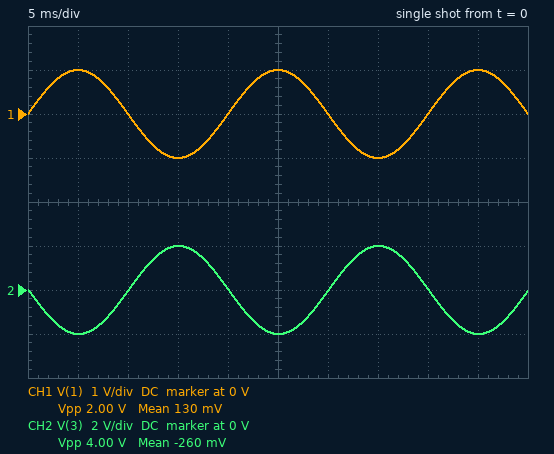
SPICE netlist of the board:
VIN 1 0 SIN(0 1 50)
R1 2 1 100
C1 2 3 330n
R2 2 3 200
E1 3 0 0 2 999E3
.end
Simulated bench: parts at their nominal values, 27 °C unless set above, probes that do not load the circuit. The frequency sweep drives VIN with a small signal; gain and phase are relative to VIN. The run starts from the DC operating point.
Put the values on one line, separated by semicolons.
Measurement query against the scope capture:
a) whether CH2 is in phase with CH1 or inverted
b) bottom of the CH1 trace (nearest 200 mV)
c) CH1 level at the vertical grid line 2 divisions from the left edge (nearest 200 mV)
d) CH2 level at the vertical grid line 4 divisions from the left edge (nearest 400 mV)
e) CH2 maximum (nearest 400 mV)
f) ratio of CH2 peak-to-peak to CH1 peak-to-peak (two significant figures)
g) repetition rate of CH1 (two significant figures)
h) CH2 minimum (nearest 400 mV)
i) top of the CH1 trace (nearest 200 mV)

inverted; -1.0 V; 0 V; 0 V; 2.0 V; 2.0; 50 Hz; -2.0 V; 1.0 V
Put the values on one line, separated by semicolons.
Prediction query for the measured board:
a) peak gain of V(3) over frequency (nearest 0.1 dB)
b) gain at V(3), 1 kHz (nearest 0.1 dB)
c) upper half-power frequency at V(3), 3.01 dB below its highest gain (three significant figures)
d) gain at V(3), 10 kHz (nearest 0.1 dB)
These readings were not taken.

6.0 dB; 5.3 dB; 2.41 kHz; -6.6 dB
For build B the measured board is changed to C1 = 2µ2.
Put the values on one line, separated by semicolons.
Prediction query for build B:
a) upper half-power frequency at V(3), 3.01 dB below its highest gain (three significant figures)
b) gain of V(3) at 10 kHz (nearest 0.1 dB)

362 Hz; -22.8 dB
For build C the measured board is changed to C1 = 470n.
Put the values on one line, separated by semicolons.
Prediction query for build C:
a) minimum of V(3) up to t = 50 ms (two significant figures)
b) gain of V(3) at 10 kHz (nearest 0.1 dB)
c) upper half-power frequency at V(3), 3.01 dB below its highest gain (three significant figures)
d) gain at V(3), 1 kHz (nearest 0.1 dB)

-2.0 V; -9.5 dB; 1.69 kHz; 4.7 dB
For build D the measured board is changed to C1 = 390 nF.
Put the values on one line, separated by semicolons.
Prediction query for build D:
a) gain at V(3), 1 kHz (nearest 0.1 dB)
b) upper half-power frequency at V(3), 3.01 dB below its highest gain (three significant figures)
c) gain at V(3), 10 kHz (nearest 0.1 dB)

5.1 dB; 2.04 kHz; -8.0 dB
